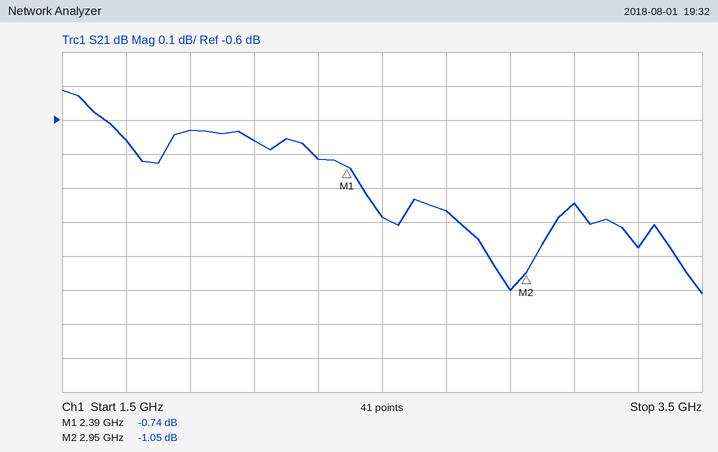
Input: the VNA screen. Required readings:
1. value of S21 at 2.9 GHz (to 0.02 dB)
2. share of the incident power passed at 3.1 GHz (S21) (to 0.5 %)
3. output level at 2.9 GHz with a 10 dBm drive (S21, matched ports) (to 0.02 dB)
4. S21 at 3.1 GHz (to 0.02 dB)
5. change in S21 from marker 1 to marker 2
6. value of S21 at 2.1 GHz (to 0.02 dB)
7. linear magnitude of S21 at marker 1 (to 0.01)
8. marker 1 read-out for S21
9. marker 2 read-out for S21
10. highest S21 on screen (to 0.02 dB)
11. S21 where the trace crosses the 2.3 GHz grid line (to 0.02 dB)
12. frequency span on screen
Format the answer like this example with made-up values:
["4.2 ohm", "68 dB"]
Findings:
["-1.10 dB", "82.5 %", "8.90 dBm", "-0.84 dB", "-0.31 dB", "-0.66 dB", "0.92", "-0.74 dB", "-1.05 dB", "-0.52 dB", "-0.72 dB", "2 GHz"]
